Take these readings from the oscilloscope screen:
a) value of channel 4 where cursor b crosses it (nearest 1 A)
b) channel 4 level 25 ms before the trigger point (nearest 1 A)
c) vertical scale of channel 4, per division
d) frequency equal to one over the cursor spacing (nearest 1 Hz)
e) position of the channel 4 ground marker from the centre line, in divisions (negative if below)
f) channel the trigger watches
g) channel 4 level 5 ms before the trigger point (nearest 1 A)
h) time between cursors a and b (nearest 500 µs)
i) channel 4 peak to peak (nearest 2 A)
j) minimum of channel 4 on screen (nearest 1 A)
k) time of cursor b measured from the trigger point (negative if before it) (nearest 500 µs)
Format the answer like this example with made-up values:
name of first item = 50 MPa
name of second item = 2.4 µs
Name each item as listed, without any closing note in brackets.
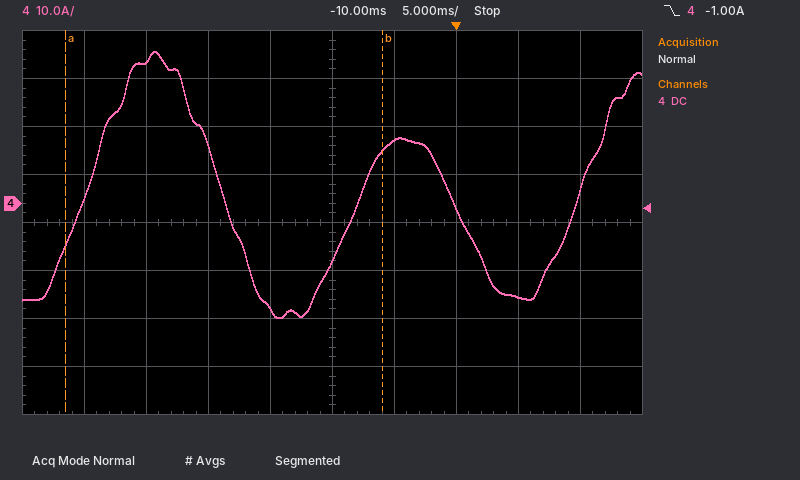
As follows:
value of channel 4 where cursor b crosses it = 11 A
channel 4 level 25 ms before the trigger point = 30 A
vertical scale of channel 4, per division = 10 A
frequency equal to one over the cursor spacing = 39 Hz
position of the channel 4 ground marker from the centre line, in divisions = +0.4 div
channel the trigger watches = channel 4
channel 4 level 5 ms before the trigger point = 13 A
time between cursors a and b = 25.5 ms
channel 4 peak to peak = 56 A
minimum of channel 4 on screen = -24 A
time of cursor b measured from the trigger point (negative if before it) = -6.0 ms
